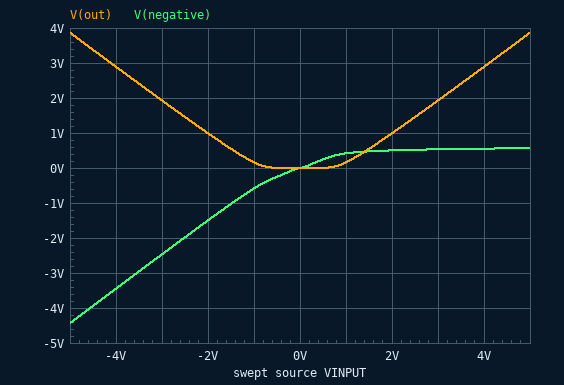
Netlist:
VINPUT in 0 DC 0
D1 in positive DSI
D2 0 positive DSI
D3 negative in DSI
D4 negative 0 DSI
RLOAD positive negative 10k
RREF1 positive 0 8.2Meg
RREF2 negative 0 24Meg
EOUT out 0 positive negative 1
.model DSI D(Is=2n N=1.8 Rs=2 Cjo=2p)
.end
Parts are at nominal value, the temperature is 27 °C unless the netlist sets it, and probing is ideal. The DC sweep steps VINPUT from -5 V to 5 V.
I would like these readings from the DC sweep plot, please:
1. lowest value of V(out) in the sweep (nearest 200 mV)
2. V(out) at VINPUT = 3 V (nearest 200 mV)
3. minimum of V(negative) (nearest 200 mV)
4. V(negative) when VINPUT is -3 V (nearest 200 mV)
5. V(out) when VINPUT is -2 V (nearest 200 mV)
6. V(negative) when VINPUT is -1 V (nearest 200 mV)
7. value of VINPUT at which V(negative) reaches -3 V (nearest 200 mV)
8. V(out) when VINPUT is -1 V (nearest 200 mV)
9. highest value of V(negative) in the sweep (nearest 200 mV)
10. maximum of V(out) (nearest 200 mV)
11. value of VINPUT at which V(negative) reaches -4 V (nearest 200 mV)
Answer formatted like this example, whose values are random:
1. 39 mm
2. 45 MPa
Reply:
1. 0 V
2. 2.0 V
3. -4.4 V
4. -2.4 V
5. 1.0 V
6. -600 mV
7. -3.6 V
8. 200 mV
9. 600 mV
10. 3.8 V
11. -4.6 V
